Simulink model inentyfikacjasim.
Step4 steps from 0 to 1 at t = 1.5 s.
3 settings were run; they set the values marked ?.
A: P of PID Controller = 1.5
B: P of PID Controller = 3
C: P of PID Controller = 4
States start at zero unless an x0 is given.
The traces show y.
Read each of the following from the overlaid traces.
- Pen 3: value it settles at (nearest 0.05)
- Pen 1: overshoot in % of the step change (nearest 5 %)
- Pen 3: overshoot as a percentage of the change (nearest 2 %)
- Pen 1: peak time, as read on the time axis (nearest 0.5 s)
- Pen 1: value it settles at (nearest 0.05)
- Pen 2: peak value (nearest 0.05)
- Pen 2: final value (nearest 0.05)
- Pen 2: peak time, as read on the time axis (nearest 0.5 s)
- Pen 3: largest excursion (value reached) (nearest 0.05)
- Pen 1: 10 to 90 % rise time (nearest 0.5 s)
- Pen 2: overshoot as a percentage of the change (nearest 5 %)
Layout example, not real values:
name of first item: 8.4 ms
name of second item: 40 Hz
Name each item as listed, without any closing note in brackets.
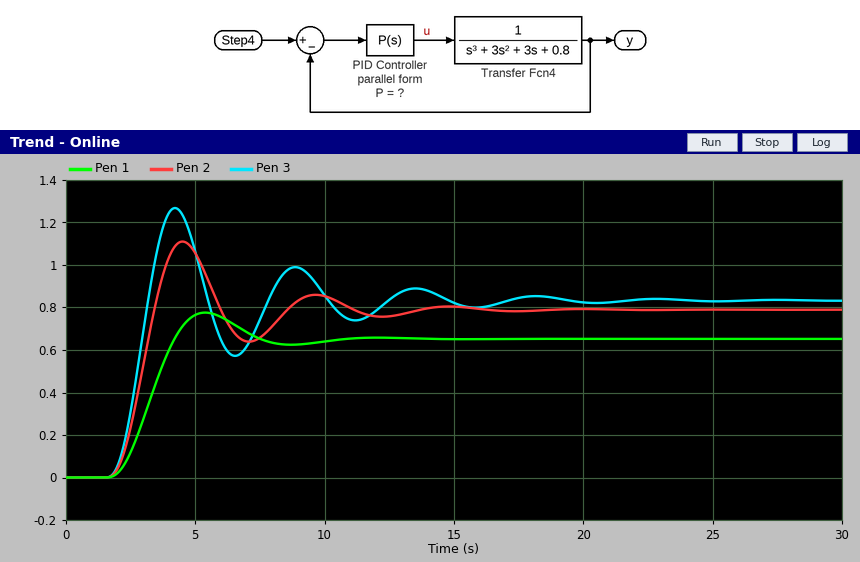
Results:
Pen 3: value it settles at: 0.85
Pen 1: overshoot in % of the step change: 20 %
Pen 3: overshoot as a percentage of the change: 52 %
Pen 1: peak time, as read on the time axis: 5.5 s
Pen 1: value it settles at: 0.65
Pen 2: peak value: 1.10
Pen 2: final value: 0.80
Pen 2: peak time, as read on the time axis: 4.5 s
Pen 3: largest excursion (value reached): 1.25
Pen 1: 10 to 90 % rise time: 1.5 s
Pen 2: overshoot as a percentage of the change: 40 %
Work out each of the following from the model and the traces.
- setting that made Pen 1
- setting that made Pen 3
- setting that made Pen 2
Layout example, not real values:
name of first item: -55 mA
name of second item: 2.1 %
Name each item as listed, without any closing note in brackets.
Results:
setting that made Pen 1: A
setting that made Pen 3: C
setting that made Pen 2: B
